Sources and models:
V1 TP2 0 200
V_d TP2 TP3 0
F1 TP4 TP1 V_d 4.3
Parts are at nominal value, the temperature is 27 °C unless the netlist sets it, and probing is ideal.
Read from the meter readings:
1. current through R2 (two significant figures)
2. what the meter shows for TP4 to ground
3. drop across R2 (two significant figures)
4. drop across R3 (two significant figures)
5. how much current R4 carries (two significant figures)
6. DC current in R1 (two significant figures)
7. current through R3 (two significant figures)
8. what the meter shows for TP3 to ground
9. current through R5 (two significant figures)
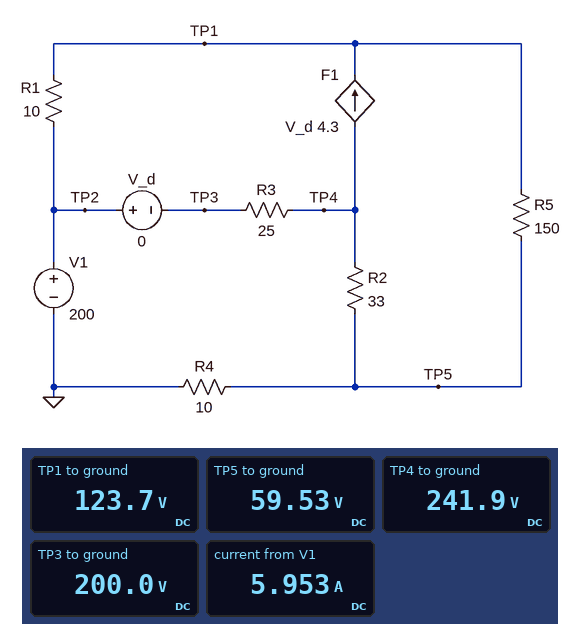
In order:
5.5 A
241.9 V
180 V
42 V
6.0 A
7.6 A
1.7 A
200.0 V
430 mA
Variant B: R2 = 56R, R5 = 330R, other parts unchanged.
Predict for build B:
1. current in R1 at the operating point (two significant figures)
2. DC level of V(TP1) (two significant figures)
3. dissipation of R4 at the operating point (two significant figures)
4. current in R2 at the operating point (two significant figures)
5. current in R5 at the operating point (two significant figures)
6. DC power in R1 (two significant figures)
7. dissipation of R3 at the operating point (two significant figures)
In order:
4.7 A
150 V
140 W
3.4 A
350 mA
220 W
26 W
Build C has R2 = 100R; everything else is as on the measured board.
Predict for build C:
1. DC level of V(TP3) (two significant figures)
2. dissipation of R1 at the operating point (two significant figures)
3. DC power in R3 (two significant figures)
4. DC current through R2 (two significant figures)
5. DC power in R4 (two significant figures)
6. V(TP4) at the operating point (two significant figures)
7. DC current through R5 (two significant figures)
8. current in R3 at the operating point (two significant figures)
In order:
200 V
110 W
8.0 W
1.9 A
78 W
210 V
920 mA
560 mA
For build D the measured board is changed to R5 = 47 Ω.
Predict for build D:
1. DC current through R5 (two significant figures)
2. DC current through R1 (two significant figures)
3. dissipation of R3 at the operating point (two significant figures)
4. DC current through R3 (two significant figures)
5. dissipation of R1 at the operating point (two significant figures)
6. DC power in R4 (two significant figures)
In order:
1.2 A
8.1 A
65 W
1.6 A
650 W
420 W
